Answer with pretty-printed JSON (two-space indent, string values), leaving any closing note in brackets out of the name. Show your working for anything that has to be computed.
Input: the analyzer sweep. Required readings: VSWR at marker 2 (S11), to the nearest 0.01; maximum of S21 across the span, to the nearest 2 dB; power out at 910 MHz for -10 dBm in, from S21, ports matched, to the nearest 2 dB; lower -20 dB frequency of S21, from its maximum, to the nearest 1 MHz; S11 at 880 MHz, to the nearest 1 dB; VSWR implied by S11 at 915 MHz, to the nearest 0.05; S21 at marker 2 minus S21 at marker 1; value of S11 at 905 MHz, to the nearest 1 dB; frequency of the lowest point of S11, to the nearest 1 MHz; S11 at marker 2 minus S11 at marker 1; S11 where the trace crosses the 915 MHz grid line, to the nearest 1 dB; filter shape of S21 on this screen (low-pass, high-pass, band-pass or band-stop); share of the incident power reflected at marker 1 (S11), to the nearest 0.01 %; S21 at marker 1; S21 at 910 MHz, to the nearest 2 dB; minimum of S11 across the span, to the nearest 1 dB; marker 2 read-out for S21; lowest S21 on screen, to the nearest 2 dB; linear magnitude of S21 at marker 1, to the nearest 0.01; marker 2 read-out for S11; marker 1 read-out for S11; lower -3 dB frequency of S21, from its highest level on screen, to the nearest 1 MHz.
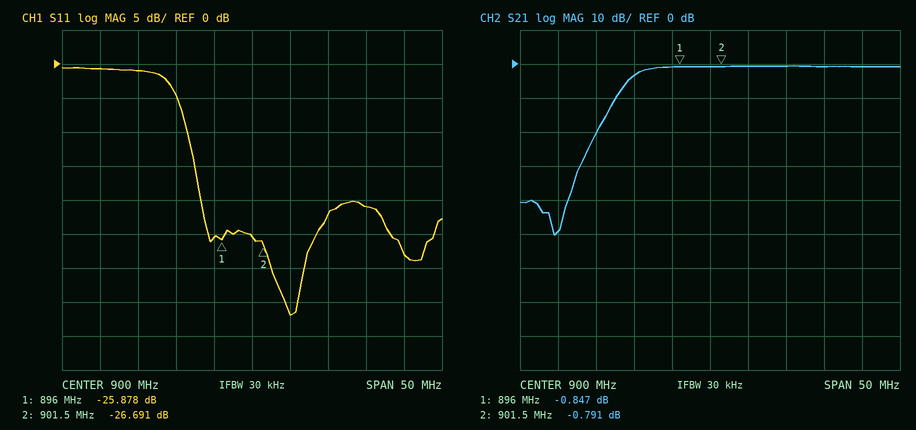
{
  "VSWR at marker 2 (S11), to the nearest 0.01": "(1 + 0.0463)/(1 − 0.0463) ≈ 1.10",
  "maximum of S21 across the span, to the nearest 2 dB": "0 dB",
  "power out at 910 MHz for -10 dBm in, from S21, ports matched, to the nearest 2 dB": "-10 dBm + (0 dB) = -10 dBm",
  "lower -20 dB frequency of S21, from its maximum, to the nearest 1 MHz": "885 MHz",
  "S11 at 880 MHz, to the nearest 1 dB": "-1 dB",
  "VSWR implied by S11 at 915 MHz, to the nearest 0.05": "|Γ| = 10^(-21/20) = 0.0891; VSWR = (1 + 0.0891)/(1 − 0.0891) ≈ 1.20",
  "S21 at marker 2 minus S21 at marker 1": "-0.791 − (-0.847) = 0.056 dB",
  "value of S11 at 905 MHz, to the nearest 1 dB": "-37 dB",
  "frequency of the lowest point of S11, to the nearest 1 MHz": "905 MHz",
  "S11 at marker 2 minus S11 at marker 1": "-26.691 − (-25.878) = -0.813 dB",
  "S11 where the trace crosses the 915 MHz grid line, to the nearest 1 dB": "-21 dB",
  "filter shape of S21 on this screen": "high-pass",
  "share of the incident power reflected at marker 1 (S11), to the nearest 0.01 %": "10^(-25.878/10) ≈ 0.26 %",
  "S21 at marker 1": "-0.847 dB",
  "S21 at 910 MHz, to the nearest 2 dB": "0 dB",
  "minimum of S11 across the span, to the nearest 1 dB": "-37 dB",
  "marker 2 read-out for S21": "-0.791 dB",
  "lowest S21 on screen, to the nearest 2 dB": "-50 dB",
  "linear magnitude of S21 at marker 1, to the nearest 0.01": "10^(-0.847/20) ≈ 0.91",
  "marker 2 read-out for S11": "-26.691 dB",
  "marker 1 read-out for S11": "-25.878 dB",
  "lower -3 dB frequency of S21, from its highest level on screen, to the nearest 1 MHz": "890 MHz"
}
